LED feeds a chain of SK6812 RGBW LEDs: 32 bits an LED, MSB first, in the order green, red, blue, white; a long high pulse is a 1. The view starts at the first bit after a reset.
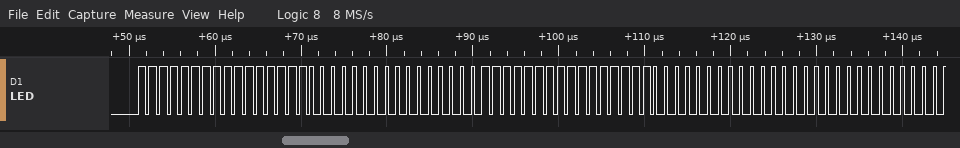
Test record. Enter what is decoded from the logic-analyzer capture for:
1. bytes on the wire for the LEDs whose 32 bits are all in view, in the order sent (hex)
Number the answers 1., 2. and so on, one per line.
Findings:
1. FF FF 00 00 FF FF 00 00
